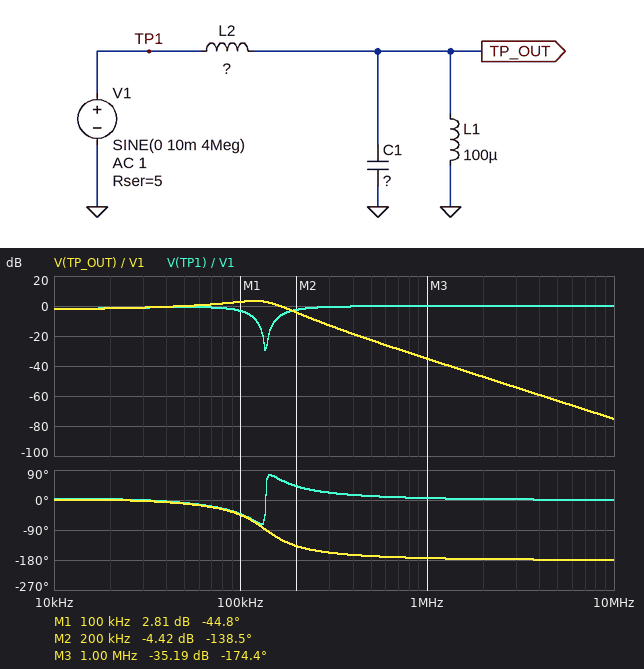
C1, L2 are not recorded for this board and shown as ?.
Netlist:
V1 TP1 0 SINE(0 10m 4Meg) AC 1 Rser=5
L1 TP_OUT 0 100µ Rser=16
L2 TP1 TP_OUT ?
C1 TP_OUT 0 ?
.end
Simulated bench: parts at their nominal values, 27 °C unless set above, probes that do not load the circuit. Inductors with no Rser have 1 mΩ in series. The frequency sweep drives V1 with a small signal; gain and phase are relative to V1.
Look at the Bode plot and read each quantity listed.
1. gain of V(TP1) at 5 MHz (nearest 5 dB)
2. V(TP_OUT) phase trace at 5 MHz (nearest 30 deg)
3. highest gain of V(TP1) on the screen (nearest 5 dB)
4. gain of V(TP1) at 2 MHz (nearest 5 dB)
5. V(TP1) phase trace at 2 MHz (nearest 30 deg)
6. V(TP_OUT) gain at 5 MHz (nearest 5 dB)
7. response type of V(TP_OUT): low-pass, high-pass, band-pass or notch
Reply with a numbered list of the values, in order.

1. 0 dB
2. -180 deg
3. 0 dB
4. 0 dB
5. 0 deg
6. -65 dB
7. low-pass
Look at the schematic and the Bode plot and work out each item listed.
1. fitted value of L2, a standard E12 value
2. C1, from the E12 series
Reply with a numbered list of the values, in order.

1. 8.2 µH
2. 180 nF
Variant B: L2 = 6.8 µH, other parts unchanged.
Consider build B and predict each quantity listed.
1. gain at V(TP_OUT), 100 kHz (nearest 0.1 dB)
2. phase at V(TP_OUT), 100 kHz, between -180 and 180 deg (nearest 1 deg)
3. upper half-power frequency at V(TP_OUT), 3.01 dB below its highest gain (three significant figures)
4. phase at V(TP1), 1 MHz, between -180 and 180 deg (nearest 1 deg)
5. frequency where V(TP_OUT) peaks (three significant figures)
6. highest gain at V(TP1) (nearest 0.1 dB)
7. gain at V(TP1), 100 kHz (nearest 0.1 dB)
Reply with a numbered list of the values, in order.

1. 2.1 dB
2. -40 deg
3. 175 kHz
4. 7 deg
5. 125 kHz
6. 0 dB
7. -2.6 dB
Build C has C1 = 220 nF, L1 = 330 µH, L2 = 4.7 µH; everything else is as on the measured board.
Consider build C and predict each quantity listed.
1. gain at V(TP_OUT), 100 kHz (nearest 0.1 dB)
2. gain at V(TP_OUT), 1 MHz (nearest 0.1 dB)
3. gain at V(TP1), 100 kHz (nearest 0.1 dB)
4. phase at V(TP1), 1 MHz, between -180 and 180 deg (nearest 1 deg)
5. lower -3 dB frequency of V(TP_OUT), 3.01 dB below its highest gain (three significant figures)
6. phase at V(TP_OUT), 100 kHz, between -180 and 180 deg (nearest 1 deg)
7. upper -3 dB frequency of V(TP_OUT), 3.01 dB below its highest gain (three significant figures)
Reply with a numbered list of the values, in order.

1. 0.9 dB
2. -32.1 dB
3. -3.5 dB
4. 10 deg
5. 2.93 kHz
6. -48 deg
7. 181 kHz
